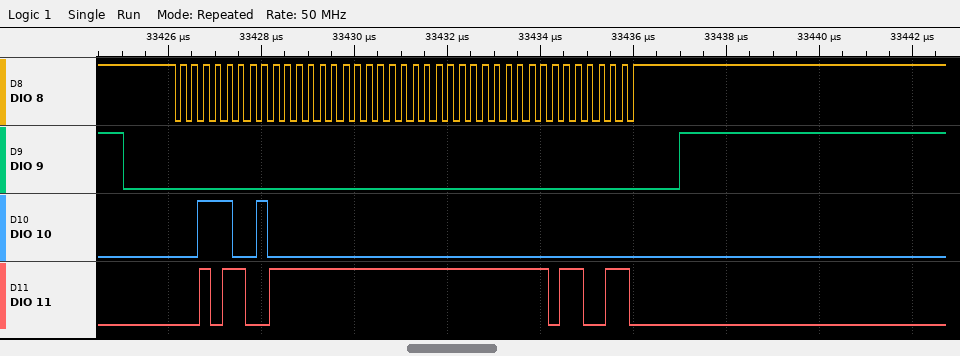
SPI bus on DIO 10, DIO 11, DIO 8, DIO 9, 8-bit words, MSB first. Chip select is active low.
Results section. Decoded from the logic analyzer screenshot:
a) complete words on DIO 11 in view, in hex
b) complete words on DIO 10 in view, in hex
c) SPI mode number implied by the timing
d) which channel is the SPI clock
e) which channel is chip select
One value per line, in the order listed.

2C, FF, FF, FF, 66
39, 00, 00, 00, 00
3
DIO 8
DIO 9
